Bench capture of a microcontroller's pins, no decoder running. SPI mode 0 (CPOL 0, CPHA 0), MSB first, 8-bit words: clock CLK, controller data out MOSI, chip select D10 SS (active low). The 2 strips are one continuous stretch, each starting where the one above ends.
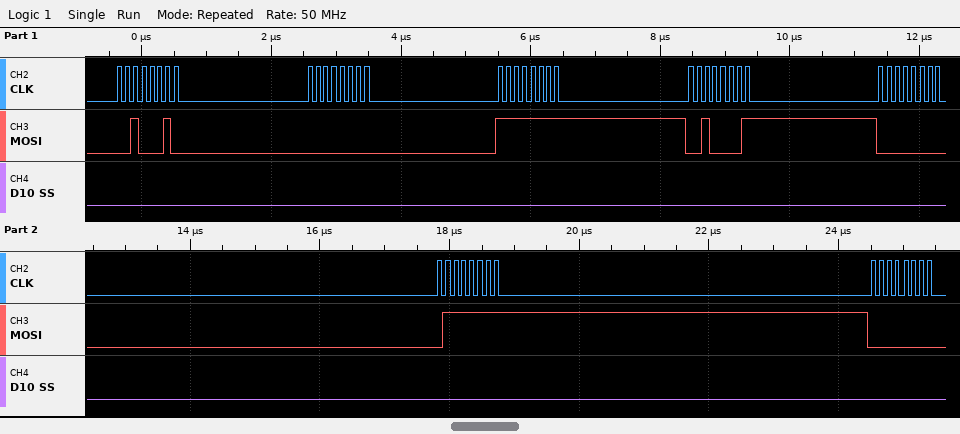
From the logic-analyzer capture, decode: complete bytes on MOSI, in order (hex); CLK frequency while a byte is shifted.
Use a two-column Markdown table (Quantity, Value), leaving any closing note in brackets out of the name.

| Quantity | Value |
|---|---|
| complete bytes on MOSI, in order | 22 00 FF 21 00 7F 00 |
| CLK frequency while a byte is shifted | 8 MHz |
